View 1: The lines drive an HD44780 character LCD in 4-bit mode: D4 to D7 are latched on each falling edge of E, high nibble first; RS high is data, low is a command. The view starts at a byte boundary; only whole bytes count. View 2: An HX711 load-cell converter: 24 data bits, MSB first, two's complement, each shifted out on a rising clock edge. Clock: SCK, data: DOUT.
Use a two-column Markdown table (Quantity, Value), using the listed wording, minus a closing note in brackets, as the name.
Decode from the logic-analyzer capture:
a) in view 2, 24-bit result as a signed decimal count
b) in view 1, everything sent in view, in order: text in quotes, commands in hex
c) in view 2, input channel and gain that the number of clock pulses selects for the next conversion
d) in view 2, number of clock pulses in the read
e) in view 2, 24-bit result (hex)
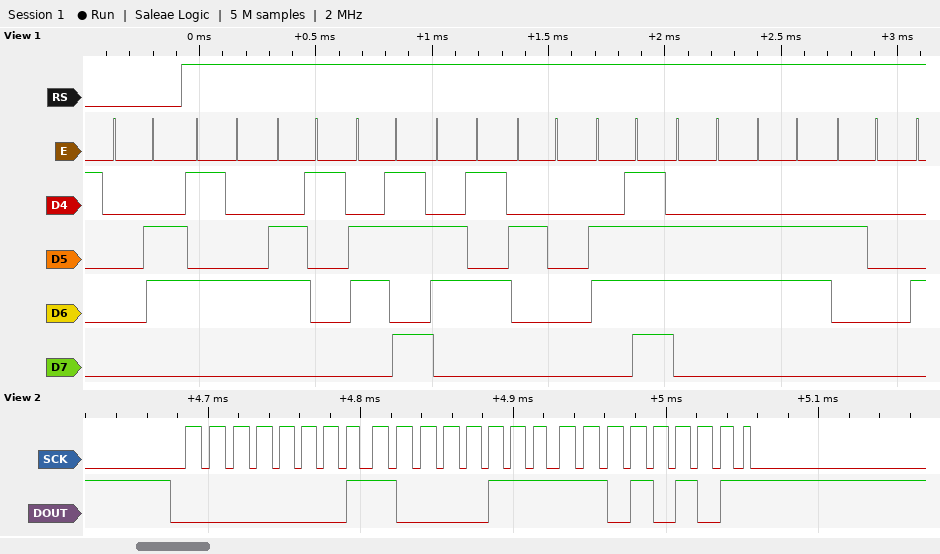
| Quantity | Value |
|---|---|
| in view 2, 24-bit result as a signed decimal count | 100309 |
| in view 1, everything sent in view, in order: text in quotes, commands in hex | 0x06 "Take off " |
| in view 2, input channel and gain that the number of clock pulses selects for the next conversion | channel A, gain 128 |
| in view 2, number of clock pulses in the read | 25 |
| in view 2, 24-bit result | 0x0187D5 |
